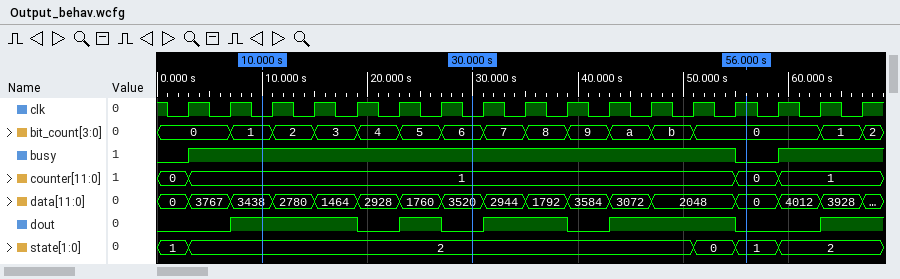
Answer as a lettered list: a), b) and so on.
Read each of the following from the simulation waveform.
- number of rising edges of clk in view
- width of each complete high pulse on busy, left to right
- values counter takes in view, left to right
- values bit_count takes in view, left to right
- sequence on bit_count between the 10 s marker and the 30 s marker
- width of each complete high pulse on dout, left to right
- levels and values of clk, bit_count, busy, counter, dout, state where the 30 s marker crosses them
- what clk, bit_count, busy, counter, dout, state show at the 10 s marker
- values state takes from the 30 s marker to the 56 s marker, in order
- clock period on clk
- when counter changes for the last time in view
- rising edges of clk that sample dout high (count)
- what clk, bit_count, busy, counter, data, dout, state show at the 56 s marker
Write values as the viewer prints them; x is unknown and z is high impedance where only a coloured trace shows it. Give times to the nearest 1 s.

a) 17
b) 52 s
c) 0, 1, 0, 1
d) 0, 1, 2, 3, 4, 5, 6, 7, 8, 9, a, b, 0, 1, 2
e) 1, 2, 3, 4, 5, 6
f) 12 s, 4 s, 8 s, 12 s
g) clk=0, bit_count=6, busy=1, counter=1, dout=0, state=2
h) clk=0, bit_count=1, busy=1, counter=1, dout=1, state=2
i) 2, 0, 1
j) 4 s
k) 59 s
l) 10
m) clk=1, bit_count=0, busy=0, counter=0, data=0, dout=0, state=1
